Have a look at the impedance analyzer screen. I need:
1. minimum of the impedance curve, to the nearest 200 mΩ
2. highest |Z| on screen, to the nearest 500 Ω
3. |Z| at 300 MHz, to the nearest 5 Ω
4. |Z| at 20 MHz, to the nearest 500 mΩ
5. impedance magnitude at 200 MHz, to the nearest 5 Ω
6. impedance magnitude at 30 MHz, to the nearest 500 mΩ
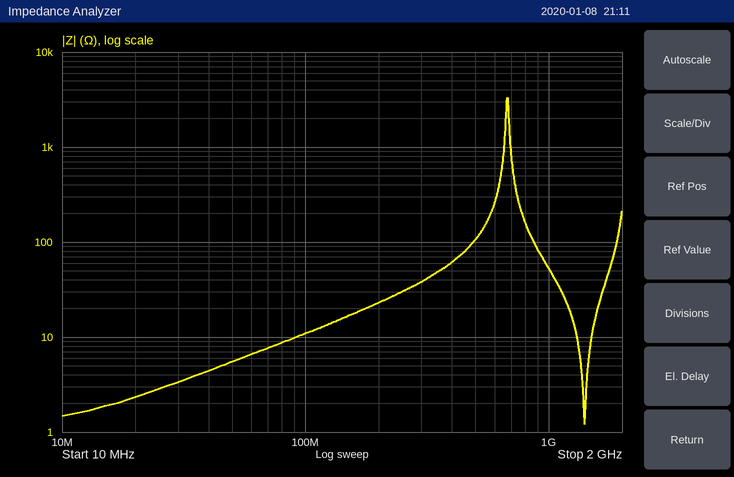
1.2 Ω
3.5 kΩ
40 Ω
2.5 Ω
25 Ω
3.5 Ω
